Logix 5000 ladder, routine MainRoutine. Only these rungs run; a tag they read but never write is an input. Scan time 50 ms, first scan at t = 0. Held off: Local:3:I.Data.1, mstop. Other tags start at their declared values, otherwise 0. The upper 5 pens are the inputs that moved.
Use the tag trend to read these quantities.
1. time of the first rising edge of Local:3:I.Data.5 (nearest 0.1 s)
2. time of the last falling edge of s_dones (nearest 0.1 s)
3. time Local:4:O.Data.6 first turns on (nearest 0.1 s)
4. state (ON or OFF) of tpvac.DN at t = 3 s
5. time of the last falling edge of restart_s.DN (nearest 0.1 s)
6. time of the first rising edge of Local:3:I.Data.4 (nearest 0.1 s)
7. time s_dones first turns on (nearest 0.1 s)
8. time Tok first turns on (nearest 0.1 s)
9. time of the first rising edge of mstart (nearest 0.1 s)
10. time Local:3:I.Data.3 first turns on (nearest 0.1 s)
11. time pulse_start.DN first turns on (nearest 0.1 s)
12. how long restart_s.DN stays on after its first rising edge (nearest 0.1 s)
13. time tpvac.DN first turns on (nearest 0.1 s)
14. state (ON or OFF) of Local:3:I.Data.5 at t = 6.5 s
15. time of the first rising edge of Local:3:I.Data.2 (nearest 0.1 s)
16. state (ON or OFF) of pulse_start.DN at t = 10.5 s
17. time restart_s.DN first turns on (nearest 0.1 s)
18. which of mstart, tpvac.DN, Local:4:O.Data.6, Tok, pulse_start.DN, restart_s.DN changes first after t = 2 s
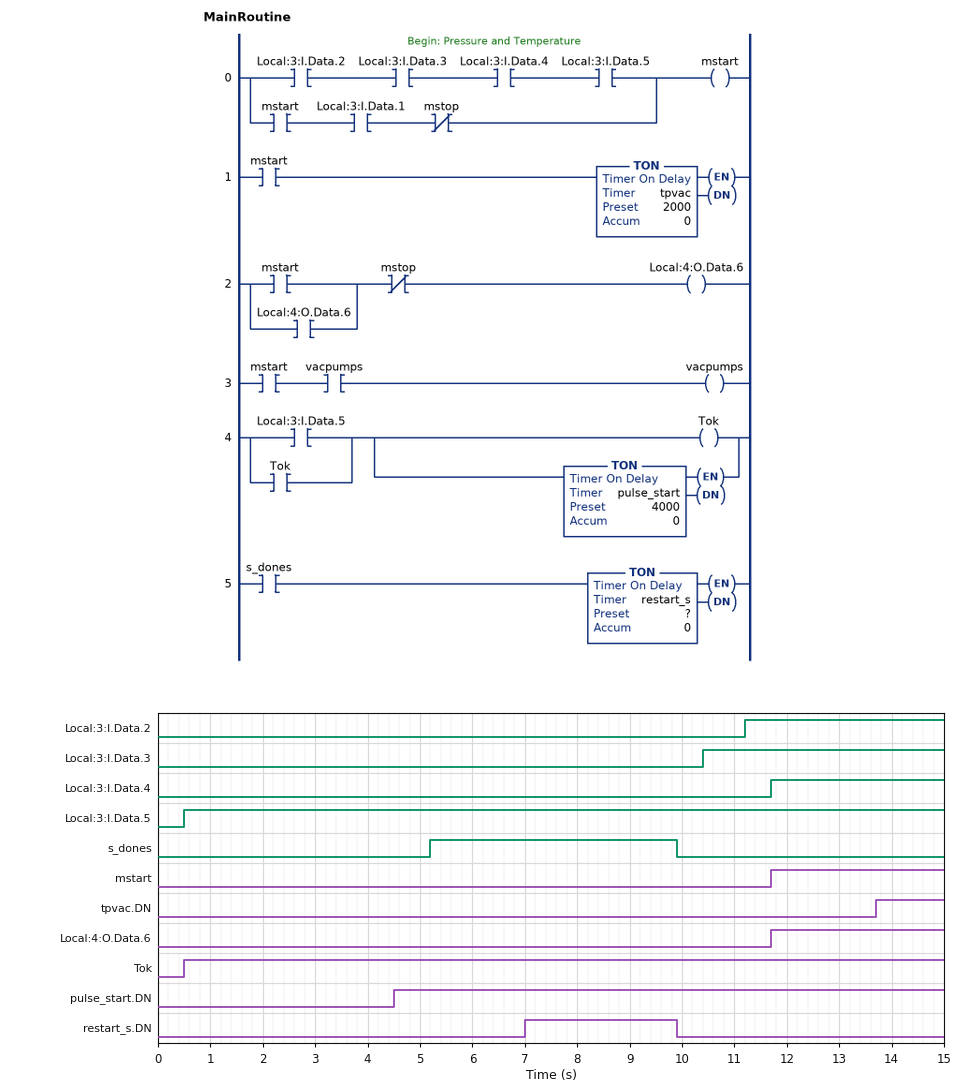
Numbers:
0.5 s
9.9 s
11.7 s
OFF
9.9 s
11.7 s
5.2 s
0.5 s
11.7 s
10.4 s
4.5 s
2.9 s
13.7 s
ON
11.2 s
ON
7.0 s
pulse_start.DN
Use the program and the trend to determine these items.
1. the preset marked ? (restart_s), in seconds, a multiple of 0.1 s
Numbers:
1.8 s
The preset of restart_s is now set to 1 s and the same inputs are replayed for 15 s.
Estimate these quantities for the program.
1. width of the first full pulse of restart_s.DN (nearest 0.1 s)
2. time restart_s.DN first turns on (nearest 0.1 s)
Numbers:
3.7 s
6.2 s
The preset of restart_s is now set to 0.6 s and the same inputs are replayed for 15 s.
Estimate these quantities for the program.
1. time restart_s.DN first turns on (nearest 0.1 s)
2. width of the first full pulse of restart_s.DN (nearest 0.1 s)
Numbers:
5.8 s
4.1 s
